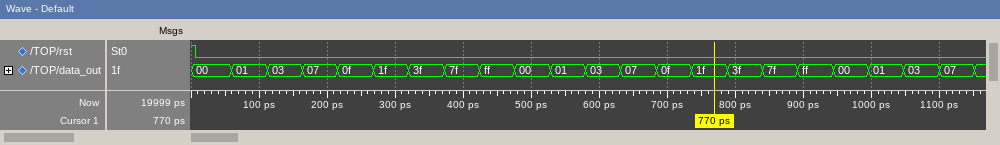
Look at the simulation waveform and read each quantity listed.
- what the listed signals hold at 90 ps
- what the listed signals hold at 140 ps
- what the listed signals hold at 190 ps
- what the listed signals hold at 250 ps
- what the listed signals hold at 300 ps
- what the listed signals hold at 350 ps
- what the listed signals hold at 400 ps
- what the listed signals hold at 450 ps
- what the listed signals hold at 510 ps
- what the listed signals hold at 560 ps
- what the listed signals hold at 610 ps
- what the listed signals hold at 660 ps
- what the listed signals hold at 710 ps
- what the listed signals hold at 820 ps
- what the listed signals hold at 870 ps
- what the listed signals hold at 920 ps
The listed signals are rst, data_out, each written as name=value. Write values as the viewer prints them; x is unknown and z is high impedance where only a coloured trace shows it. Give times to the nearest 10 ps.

rst=0, data_out=01
rst=0, data_out=03
rst=0, data_out=07
rst=0, data_out=0f
rst=0, data_out=1f
rst=0, data_out=3f
rst=0, data_out=7f
rst=0, data_out=ff
rst=0, data_out=00
rst=0, data_out=01
rst=0, data_out=03
rst=0, data_out=07
rst=0, data_out=0f
rst=0, data_out=3f
rst=0, data_out=7f
rst=0, data_out=ff
